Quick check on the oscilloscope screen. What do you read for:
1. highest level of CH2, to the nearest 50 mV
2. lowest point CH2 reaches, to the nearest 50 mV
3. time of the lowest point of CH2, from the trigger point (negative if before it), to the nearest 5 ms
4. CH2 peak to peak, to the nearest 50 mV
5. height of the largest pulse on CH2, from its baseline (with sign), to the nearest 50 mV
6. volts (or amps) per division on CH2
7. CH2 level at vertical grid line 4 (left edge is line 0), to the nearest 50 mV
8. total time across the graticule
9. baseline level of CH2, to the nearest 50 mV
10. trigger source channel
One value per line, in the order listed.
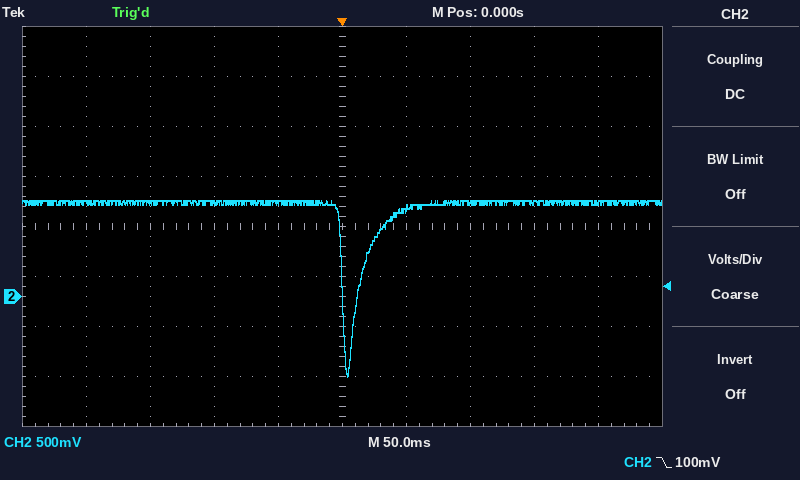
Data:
950 mV
-800 mV
+5 ms
1.75 V
-1.75 V
500 mV
950 mV
500 ms
950 mV
CH2
